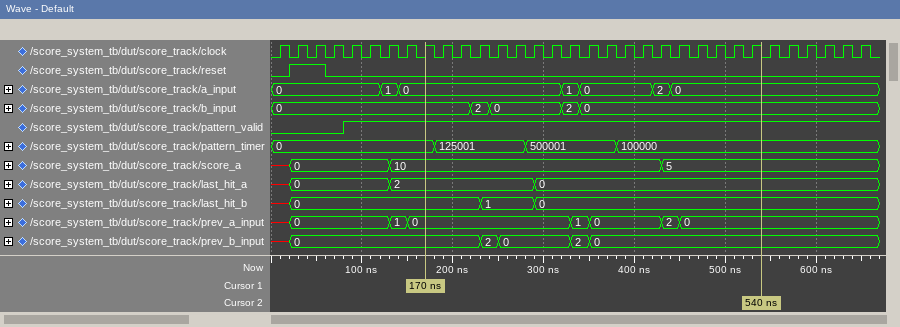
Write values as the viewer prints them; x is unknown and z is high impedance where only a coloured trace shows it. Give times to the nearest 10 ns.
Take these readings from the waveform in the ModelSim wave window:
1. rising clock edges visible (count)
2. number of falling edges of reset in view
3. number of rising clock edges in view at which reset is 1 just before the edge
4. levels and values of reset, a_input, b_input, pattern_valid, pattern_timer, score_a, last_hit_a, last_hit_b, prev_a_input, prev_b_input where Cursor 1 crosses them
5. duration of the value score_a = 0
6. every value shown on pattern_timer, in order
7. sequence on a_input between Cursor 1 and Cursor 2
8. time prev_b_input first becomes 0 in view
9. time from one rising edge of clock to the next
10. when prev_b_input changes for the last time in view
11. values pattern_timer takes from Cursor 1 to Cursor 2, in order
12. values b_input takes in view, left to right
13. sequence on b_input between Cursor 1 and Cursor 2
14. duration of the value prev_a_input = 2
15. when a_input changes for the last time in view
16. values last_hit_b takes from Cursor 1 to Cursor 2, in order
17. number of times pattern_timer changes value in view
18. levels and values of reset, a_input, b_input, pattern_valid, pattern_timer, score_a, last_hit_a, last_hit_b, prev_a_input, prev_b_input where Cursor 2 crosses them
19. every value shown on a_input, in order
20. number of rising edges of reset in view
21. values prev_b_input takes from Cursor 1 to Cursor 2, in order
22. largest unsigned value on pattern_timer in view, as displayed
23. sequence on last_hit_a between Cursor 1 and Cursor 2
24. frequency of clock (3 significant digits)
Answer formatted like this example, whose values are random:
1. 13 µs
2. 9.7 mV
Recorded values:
1. 33
2. 1
3. 2
4. reset=0, a_input=0, b_input=0, pattern_valid=1, pattern_timer=0, score_a=10, last_hit_a=2, last_hit_b=0, prev_a_input=0, prev_b_input=0
5. 110 ns
6. 0, 125001, 500001, 100000
7. 0, 1, 0, 2, 0
8. 20 ns
9. 20 ns
10. 350 ns
11. 0, 125001, 500001, 100000
12. 0, 2, 0, 2, 0
13. 0, 2, 0, 2, 0
14. 20 ns
15. 440 ns
16. 0, 1, 0
17. 3
18. reset=0, a_input=0, b_input=0, pattern_valid=1, pattern_timer=100000, score_a=5, last_hit_a=0, last_hit_b=0, prev_a_input=0, prev_b_input=0
19. 0, 1, 0, 1, 0, 2, 0
20. 1
21. 0, 2, 0, 2, 0
22. 500001
23. 2, 0
24. 50.0 MHz
